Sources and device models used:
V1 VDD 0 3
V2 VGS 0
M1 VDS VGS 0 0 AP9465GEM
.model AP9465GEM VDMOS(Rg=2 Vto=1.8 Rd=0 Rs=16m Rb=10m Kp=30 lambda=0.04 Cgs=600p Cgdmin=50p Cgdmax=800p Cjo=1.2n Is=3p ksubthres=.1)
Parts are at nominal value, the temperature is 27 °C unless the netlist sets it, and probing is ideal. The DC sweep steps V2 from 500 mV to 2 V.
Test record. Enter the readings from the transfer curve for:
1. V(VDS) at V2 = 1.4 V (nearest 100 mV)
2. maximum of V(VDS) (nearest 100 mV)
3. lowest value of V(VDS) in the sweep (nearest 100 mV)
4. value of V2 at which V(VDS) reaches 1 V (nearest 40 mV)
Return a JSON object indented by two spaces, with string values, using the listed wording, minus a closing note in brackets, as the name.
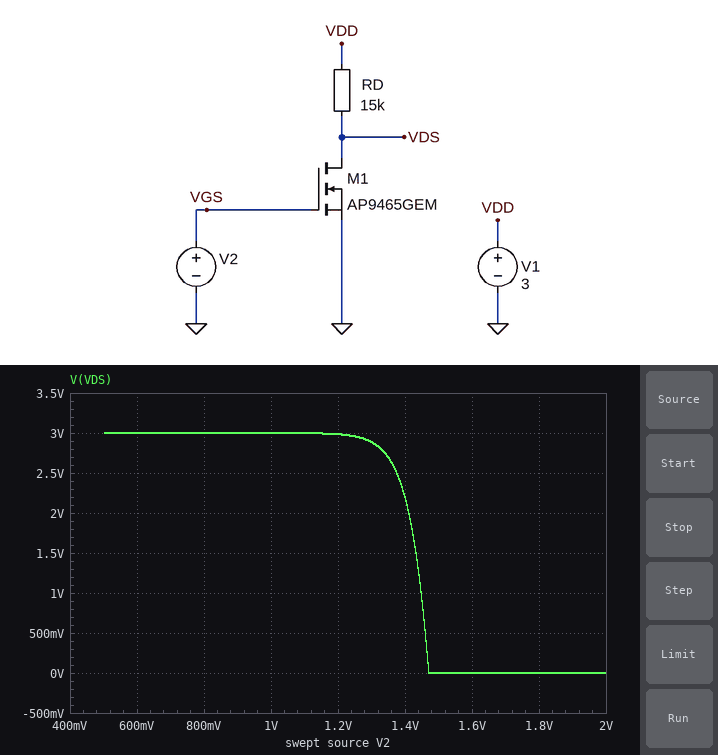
{
  "V(VDS) at V2 = 1.4 V": "2.2 V",
  "maximum of V(VDS)": "3.0 V",
  "lowest value of V(VDS) in the sweep": "0 V",
  "value of V2 at which V(VDS) reaches 1 V": "1.44 V"
}
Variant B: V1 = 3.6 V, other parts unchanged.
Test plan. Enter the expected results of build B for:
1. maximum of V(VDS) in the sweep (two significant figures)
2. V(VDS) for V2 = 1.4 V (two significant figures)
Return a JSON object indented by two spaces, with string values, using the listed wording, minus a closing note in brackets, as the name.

{
  "maximum of V(VDS) in the sweep": "3.6 V",
  "V(VDS) for V2 = 1.4 V": "2.8 V"
}
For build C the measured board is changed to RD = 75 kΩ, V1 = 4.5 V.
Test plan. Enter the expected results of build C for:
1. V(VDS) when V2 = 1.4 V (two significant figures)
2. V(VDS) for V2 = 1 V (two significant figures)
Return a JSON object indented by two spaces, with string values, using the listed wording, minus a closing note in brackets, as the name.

{
  "V(VDS) when V2 = 1.4 V": "690 mV",
  "V(VDS) for V2 = 1 V": "4.5 V"
}
